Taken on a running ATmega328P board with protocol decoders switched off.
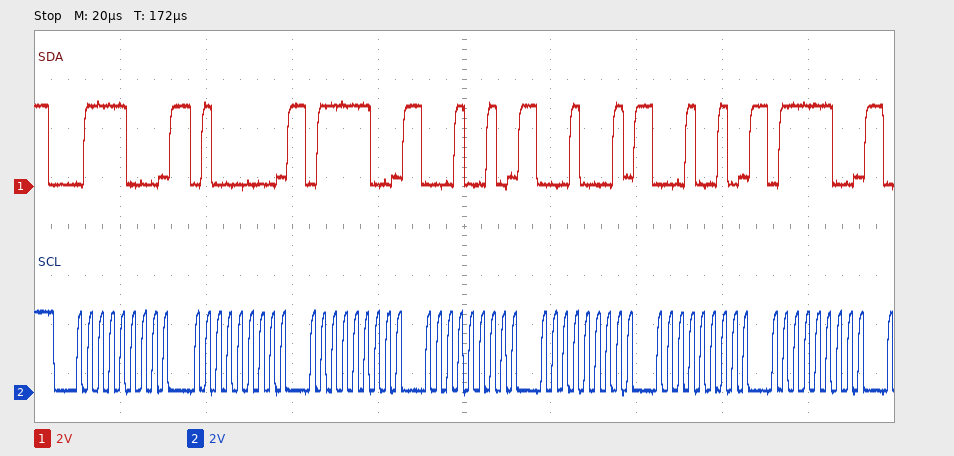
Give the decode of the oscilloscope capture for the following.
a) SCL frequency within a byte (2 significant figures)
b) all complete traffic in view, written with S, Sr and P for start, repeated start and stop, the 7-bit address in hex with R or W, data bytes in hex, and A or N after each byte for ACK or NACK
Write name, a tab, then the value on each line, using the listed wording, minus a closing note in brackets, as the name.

SCL frequency within a byte	400 kHz
all complete traffic in view, written with S, Sr and P for start, repeated start and stop, the 7-bit address in hex with R or W, data bytes in hex, and A or N after each byte for ACK or NACK	S 3CW A 40 A 7C A 12 A 11 A 12 A 7C A
